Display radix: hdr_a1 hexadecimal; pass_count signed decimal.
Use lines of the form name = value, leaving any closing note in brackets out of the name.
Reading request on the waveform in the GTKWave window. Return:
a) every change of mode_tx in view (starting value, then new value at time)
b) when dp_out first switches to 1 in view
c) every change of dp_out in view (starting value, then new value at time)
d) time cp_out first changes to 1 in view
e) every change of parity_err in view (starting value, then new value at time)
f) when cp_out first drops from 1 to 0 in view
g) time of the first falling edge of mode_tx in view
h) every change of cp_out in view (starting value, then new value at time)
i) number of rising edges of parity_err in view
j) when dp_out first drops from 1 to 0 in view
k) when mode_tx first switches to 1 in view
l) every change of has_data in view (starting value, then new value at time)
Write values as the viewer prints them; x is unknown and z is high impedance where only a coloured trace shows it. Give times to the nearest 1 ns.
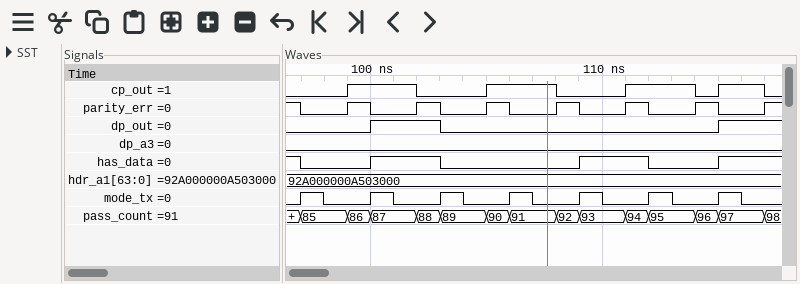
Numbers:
every change of mode_tx in view = 0, 1 at 97 ns, 0 at 98 ns, 1 at 100 ns, 0 at 101 ns, 1 at 103 ns, 0 at 104 ns, 1 at 106 ns, 0 at 107 ns, 1 at 109 ns, 0 at 110 ns, 1 at 112 ns, 0 at 113 ns, 1 at 115 ns, 0 at 116 ns
when dp_out first switches to 1 in view = 100 ns
every change of dp_out in view = 0, 1 at 100 ns, 0 at 103 ns, 1 at 115 ns
time cp_out first changes to 1 in view = 99 ns
every change of parity_err in view = 1, 0 at 97 ns, 1 at 99 ns, 0 at 100 ns, 1 at 102 ns, 0 at 103 ns, 1 at 105 ns, 0 at 106 ns, 1 at 108 ns, 0 at 109 ns, 1 at 111 ns, 0 at 112 ns, 1 at 114 ns, 0 at 115 ns, 1 at 117 ns
when cp_out first drops from 1 to 0 in view = 102 ns
time of the first falling edge of mode_tx in view = 98 ns
every change of cp_out in view = 0, 1 at 99 ns, 0 at 102 ns, 1 at 105 ns, 0 at 108 ns, 1 at 111 ns, 0 at 114 ns, 1 at 115 ns, 0 at 117 ns
number of rising edges of parity_err in view = 7
when dp_out first drops from 1 to 0 in view = 103 ns
when mode_tx first switches to 1 in view = 97 ns
every change of has_data in view = 1, 0 at 97 ns, 1 at 100 ns, 0 at 103 ns, 1 at 109 ns, 0 at 112 ns, 1 at 115 ns
